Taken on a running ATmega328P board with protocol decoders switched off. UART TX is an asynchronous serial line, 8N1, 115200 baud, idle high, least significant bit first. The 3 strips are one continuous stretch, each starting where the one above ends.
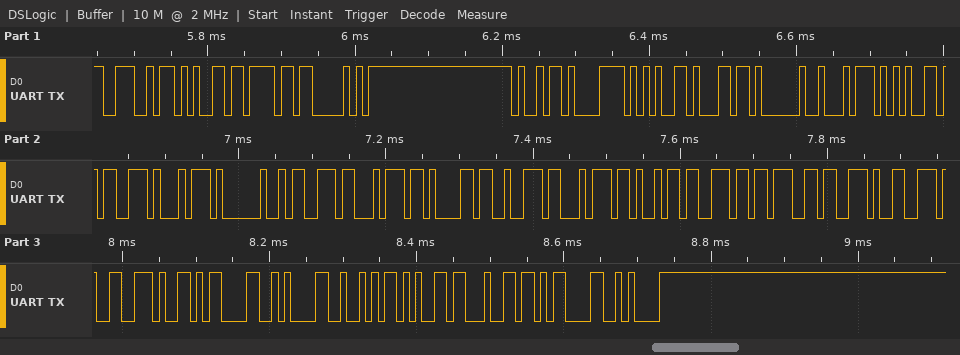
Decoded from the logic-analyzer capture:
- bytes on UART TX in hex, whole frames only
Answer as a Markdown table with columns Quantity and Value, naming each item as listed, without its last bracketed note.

| Quantity | Value |
|---|---|
| bytes on UART TX in hex, whole frames only | 4E 65 6F 50 69 78 65 6C 20 74 65 73 74 20 73 74 61 72 74 69 6E 67 2E 2E 2E 0D 0A 52 65 64 0D 0A |
